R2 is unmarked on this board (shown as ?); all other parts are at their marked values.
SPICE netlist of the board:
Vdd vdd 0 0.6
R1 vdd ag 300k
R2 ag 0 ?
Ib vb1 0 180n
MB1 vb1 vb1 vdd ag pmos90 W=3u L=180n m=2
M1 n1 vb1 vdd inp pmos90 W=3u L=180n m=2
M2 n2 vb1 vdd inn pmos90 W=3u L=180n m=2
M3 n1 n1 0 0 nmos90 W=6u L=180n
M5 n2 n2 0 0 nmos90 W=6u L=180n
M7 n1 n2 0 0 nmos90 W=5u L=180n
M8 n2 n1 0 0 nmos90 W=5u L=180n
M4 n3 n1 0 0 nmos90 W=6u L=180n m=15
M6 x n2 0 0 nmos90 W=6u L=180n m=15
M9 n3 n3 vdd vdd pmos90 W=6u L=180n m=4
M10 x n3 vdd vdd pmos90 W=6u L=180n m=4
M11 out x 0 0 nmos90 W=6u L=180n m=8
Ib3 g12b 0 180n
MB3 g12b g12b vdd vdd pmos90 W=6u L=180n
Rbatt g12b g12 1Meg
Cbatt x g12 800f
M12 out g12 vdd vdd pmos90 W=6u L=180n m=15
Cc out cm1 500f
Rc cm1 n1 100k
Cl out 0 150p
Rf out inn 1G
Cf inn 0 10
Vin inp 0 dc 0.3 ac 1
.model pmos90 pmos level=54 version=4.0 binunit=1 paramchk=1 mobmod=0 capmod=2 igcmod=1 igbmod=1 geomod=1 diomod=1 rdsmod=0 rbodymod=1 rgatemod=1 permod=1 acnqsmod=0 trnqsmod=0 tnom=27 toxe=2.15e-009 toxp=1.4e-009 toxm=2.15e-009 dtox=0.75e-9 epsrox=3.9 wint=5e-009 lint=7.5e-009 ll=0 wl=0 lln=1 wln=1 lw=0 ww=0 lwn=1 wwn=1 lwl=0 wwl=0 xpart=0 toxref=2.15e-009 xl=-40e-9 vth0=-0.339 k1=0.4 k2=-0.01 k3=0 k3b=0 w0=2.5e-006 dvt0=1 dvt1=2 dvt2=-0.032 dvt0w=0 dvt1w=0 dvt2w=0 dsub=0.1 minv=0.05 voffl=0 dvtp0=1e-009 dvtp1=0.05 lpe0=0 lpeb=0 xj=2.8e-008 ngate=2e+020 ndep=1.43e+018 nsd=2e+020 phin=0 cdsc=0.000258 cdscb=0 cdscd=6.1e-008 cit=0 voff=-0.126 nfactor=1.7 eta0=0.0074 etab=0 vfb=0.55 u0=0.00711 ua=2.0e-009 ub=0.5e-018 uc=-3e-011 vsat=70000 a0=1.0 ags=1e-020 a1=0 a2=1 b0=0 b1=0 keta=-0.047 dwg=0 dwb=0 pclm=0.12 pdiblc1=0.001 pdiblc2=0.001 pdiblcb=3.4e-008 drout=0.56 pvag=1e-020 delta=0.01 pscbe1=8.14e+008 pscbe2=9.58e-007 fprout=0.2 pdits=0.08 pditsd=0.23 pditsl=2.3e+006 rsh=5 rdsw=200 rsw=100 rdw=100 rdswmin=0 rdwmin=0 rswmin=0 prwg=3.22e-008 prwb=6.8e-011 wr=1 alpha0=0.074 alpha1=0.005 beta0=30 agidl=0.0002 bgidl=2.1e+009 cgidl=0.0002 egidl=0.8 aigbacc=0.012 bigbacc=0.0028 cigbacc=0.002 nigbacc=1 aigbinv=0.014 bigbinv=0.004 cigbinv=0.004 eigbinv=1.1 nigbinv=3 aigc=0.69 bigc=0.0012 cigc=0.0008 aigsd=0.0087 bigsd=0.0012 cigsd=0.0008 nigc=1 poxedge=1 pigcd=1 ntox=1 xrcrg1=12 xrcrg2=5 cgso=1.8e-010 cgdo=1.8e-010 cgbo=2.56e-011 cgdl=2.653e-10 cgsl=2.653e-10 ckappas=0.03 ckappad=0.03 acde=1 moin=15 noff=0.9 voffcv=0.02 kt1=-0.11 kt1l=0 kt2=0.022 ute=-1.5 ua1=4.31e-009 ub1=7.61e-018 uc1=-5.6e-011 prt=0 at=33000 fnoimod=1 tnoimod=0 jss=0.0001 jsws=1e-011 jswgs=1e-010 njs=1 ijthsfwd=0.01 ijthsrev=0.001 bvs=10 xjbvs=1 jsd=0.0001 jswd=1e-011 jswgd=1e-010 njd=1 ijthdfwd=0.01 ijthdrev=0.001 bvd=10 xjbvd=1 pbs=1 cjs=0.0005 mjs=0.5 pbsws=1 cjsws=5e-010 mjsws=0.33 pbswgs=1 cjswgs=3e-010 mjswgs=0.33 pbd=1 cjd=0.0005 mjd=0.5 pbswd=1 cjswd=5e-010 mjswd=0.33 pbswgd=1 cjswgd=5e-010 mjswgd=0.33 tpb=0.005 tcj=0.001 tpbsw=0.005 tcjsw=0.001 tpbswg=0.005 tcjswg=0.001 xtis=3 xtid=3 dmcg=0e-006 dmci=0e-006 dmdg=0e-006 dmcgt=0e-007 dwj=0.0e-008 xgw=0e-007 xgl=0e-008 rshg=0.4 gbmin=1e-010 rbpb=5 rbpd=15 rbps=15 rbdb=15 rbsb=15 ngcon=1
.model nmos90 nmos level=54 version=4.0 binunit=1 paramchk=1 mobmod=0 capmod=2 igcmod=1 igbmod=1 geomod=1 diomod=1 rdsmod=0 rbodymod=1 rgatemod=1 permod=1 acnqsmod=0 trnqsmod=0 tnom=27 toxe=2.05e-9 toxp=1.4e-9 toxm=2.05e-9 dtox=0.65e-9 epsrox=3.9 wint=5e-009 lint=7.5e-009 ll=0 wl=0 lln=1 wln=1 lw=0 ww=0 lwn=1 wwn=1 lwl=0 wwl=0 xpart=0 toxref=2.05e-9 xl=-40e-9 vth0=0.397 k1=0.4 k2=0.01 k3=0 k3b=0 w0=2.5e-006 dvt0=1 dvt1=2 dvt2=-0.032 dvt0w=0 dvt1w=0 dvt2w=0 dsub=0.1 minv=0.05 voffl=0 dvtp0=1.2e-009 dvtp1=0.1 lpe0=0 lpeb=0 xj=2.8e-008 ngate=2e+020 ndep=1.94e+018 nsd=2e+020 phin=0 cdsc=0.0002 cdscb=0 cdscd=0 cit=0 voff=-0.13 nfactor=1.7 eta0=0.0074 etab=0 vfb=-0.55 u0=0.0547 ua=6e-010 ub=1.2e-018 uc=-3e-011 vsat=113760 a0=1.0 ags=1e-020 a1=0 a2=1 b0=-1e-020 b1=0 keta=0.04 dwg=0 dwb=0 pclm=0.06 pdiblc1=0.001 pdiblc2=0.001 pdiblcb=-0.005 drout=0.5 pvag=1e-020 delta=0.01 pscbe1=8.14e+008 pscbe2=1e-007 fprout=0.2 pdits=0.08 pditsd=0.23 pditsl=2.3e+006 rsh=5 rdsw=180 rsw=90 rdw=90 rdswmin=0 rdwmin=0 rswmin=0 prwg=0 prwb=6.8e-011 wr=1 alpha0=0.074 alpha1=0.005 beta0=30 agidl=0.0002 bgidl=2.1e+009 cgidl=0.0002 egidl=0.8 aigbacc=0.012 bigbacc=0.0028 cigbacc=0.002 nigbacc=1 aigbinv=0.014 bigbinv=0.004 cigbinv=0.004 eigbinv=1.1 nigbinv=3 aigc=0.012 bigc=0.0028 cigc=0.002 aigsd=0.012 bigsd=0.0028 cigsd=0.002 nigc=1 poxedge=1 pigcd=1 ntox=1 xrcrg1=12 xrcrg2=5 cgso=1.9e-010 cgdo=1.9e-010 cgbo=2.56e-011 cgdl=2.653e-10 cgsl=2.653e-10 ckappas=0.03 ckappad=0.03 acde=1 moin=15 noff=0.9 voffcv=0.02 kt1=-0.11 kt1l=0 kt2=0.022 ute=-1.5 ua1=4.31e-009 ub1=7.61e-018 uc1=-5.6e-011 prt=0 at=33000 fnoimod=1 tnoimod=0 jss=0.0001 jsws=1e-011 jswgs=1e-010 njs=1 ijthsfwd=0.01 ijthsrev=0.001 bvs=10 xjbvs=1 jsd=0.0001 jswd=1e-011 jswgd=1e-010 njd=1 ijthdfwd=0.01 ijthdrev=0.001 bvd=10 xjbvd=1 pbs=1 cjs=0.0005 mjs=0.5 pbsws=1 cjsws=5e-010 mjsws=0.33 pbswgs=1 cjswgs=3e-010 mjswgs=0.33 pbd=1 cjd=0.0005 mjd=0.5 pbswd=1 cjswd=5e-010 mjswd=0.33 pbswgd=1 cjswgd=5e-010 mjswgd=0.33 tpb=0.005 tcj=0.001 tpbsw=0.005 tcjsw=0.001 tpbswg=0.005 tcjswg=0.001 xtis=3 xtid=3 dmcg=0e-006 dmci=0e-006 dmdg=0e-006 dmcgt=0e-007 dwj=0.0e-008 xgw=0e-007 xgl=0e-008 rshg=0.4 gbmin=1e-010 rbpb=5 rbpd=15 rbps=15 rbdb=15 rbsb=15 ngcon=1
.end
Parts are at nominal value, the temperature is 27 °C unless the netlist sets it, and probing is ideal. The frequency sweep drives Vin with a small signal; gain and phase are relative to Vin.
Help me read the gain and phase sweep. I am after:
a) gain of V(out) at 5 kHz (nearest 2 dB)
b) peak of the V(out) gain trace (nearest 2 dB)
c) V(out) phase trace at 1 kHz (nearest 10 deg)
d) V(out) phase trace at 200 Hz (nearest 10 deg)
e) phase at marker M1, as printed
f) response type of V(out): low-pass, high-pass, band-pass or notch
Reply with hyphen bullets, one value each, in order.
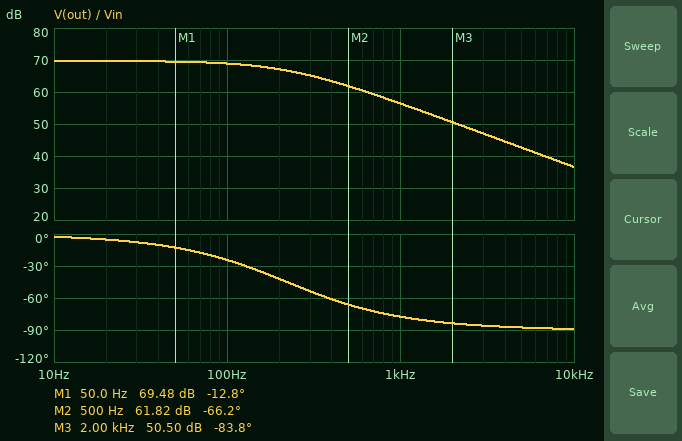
- 42 dB
- 70 dB
- -80 deg
- -40 deg
- -12.8 deg
- low-pass
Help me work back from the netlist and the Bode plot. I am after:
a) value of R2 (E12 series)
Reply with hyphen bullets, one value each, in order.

- 680 kΩ
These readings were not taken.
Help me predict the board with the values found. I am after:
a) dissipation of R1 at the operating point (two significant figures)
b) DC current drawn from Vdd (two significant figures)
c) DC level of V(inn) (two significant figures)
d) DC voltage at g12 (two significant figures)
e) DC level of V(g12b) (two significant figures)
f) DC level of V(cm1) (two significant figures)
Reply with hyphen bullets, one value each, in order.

- 110 nW
- 11 µA
- 300 mV
- 410 mV
- 410 mV
- 150 mV
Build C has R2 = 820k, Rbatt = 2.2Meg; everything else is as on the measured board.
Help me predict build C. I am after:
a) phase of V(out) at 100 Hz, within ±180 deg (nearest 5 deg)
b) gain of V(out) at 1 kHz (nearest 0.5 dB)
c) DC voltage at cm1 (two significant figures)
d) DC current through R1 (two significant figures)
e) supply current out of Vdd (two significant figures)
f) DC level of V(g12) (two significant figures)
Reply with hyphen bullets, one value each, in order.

- -20 deg
- 57.0 dB
- 160 mV
- 540 nA
- 12 µA
- 410 mV
